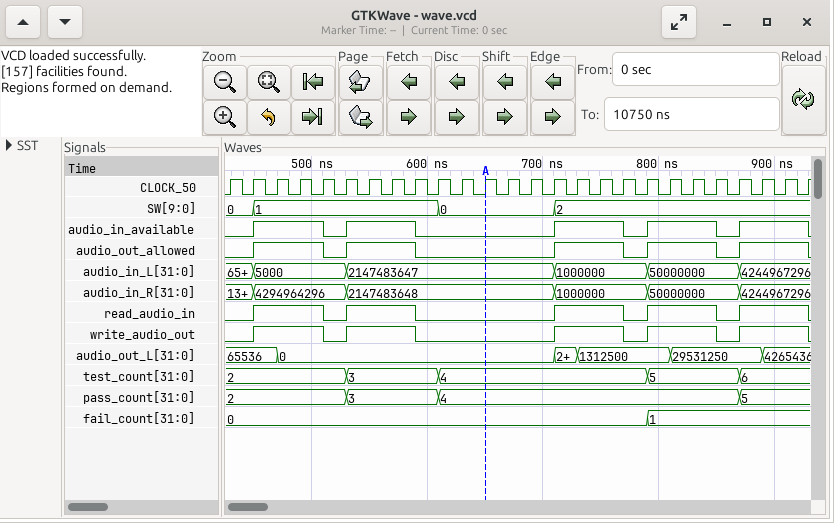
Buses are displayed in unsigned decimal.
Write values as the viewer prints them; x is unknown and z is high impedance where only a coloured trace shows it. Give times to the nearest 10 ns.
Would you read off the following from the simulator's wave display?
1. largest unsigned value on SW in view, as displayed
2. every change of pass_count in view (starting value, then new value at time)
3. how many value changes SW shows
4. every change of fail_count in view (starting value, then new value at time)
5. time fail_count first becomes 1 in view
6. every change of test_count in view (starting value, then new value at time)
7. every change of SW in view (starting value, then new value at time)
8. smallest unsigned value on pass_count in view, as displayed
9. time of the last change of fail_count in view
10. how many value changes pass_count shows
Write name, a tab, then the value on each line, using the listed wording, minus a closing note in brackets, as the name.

largest unsigned value on SW in view, as displayed	2
every change of pass_count in view	2, 3 at 530 ns, 4 at 610 ns, 5 at 870 ns
how many value changes SW shows	3
every change of fail_count in view	0, 1 at 790 ns
time fail_count first becomes 1 in view	790 ns
every change of test_count in view	2, 3 at 530 ns, 4 at 610 ns, 5 at 790 ns, 6 at 870 ns
every change of SW in view	0, 1 at 450 ns, 0 at 610 ns, 2 at 710 ns
smallest unsigned value on pass_count in view, as displayed	2
time of the last change of fail_count in view	790 ns
how many value changes pass_count shows	3
